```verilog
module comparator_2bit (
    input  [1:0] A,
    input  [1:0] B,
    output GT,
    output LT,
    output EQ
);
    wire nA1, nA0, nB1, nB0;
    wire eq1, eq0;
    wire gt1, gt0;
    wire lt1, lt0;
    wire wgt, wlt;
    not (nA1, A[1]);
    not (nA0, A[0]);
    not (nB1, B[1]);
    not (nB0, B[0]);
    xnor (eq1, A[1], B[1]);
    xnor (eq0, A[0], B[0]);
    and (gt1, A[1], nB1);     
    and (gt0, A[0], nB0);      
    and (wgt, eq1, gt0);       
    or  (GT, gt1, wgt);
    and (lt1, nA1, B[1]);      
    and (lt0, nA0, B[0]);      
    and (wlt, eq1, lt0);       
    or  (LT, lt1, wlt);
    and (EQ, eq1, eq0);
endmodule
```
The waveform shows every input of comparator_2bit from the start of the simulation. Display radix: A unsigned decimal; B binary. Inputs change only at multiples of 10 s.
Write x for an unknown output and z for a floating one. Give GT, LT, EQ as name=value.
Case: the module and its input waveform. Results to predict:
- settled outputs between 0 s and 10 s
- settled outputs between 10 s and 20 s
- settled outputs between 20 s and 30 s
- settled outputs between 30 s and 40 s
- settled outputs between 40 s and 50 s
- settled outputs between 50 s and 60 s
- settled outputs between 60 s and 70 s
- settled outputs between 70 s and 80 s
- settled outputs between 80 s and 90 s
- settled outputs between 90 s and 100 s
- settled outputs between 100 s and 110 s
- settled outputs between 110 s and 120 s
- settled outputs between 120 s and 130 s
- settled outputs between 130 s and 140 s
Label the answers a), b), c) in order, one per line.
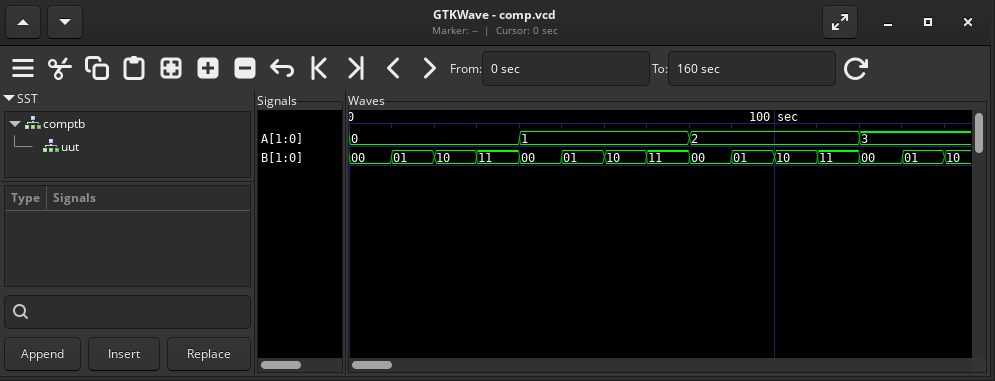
a) GT=0, LT=0, EQ=1
b) GT=0, LT=1, EQ=0
c) GT=0, LT=1, EQ=0
d) GT=0, LT=1, EQ=0
e) GT=1, LT=0, EQ=0
f) GT=0, LT=0, EQ=1
g) GT=0, LT=1, EQ=0
h) GT=0, LT=1, EQ=0
i) GT=1, LT=0, EQ=0
j) GT=1, LT=0, EQ=0
k) GT=0, LT=0, EQ=1
l) GT=0, LT=1, EQ=0
m) GT=1, LT=0, EQ=0
n) GT=1, LT=0, EQ=0
